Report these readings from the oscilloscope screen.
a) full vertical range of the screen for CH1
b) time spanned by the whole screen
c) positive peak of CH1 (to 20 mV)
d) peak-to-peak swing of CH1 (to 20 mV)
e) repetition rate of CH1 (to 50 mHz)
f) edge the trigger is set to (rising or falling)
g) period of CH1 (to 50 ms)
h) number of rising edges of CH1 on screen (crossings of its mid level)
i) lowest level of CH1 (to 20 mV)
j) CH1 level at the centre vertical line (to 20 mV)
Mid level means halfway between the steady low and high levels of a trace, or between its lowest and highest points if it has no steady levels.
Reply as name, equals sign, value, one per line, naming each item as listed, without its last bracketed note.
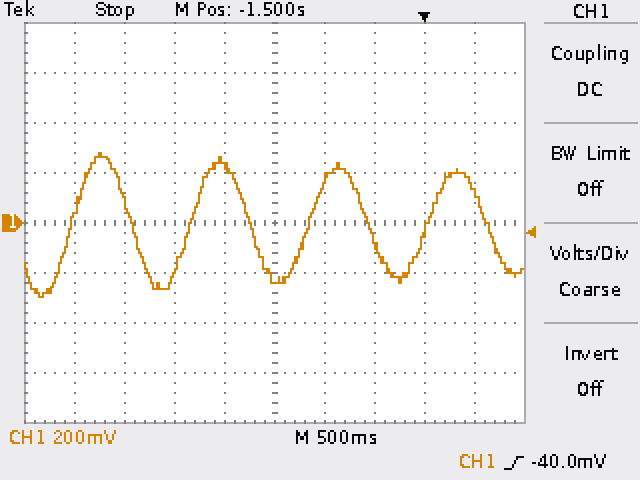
full vertical range of the screen for CH1 = 1.6 V
time spanned by the whole screen = 5 s
positive peak of CH1 = 280 mV
peak-to-peak swing of CH1 = 580 mV
repetition rate of CH1 = 850 mHz
edge the trigger is set to = rising
period of CH1 = 1.20 s
number of rising edges of CH1 on screen = 4
lowest level of CH1 = -300 mV
CH1 level at the centre vertical line = -220 mV
